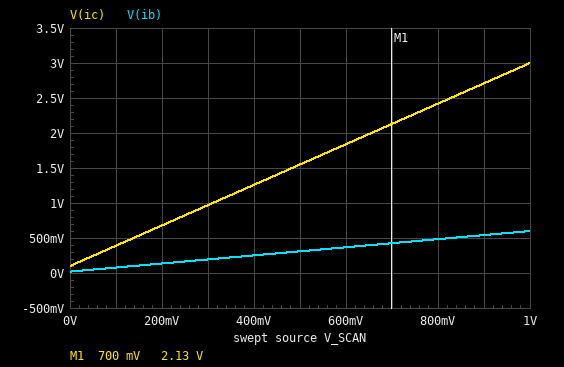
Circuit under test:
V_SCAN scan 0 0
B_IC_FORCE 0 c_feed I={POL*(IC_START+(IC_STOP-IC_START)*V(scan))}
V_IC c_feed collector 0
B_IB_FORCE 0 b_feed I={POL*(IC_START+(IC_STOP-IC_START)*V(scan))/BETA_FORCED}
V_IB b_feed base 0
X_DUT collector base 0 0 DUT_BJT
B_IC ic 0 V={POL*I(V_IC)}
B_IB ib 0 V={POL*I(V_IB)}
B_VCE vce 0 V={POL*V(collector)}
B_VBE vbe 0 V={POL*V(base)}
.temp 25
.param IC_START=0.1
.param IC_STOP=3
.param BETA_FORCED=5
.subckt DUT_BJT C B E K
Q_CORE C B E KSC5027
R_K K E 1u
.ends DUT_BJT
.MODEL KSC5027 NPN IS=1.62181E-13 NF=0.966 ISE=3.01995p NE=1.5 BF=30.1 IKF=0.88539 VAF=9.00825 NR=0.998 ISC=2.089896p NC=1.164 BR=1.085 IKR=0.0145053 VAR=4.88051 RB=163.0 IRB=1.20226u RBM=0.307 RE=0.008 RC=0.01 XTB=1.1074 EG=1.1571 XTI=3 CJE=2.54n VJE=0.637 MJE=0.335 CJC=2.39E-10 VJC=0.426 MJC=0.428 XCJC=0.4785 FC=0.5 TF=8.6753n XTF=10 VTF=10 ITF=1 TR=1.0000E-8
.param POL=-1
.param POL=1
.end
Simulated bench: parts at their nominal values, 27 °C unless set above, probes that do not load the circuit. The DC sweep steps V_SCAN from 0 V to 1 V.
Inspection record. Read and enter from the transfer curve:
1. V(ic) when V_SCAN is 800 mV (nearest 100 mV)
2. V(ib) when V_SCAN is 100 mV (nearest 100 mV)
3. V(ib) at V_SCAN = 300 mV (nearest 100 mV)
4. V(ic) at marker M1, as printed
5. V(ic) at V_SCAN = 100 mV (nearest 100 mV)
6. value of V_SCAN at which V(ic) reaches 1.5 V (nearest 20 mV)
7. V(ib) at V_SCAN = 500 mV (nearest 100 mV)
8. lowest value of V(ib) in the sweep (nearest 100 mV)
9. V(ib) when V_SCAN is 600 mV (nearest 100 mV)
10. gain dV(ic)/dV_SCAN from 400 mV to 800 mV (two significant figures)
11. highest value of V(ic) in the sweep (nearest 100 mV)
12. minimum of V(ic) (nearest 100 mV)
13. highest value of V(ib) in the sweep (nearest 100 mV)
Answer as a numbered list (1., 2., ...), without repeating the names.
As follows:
1. 2.4 V
2. 100 mV
3. 200 mV
4. 2.13 V
5. 400 mV
6. 480 mV
7. 300 mV
8. 0 V
9. 400 mV
10. 2.9 V/V
11. 3.0 V
12. 100 mV
13. 600 mV
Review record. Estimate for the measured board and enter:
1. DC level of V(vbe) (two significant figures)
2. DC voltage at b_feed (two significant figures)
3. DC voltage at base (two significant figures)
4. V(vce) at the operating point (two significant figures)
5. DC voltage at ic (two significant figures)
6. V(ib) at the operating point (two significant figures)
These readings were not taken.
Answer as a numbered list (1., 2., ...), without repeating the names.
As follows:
1. 730 mV
2. 730 mV
3. 730 mV
4. 62 mV
5. 100 mV
6. 20 mV
